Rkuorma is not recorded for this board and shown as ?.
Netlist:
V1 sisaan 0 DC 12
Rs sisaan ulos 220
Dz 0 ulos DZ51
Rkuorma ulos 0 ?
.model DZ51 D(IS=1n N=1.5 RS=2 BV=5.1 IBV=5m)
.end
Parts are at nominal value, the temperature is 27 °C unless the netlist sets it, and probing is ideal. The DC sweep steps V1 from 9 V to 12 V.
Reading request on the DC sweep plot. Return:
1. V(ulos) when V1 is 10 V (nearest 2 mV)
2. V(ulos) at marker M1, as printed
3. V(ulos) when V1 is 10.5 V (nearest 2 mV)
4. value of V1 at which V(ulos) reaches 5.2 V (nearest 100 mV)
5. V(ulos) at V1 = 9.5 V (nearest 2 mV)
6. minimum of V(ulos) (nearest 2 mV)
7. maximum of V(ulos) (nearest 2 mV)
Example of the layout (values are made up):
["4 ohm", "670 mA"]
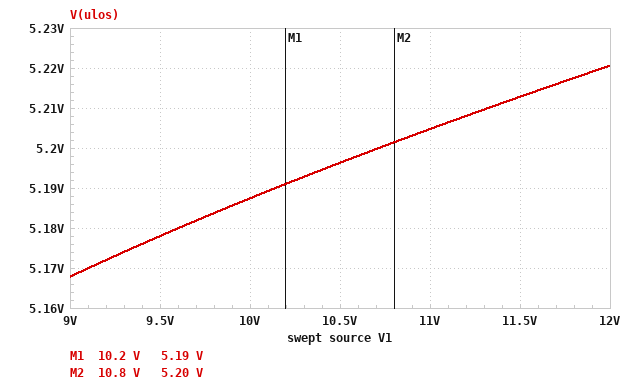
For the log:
["5.188 V", "5.19 V", "5.196 V", "10.7 V", "5.178 V", "5.168 V", "5.220 V"]
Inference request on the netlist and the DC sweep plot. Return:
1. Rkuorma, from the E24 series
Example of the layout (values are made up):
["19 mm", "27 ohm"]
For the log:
["1.5 kΩ"]
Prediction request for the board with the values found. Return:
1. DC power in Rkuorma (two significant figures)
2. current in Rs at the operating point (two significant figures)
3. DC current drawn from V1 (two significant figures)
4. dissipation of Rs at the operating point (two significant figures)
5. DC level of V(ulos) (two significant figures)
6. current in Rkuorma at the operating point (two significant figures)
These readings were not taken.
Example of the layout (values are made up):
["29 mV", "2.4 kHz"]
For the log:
["18 mW", "31 mA", "31 mA", "210 mW", "5.2 V", "3.5 mA"]
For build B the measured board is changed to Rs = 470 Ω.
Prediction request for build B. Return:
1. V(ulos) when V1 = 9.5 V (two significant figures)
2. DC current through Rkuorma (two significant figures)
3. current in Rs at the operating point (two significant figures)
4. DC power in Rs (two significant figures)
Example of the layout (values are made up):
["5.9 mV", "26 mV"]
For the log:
["5.1 V", "3.4 mA", "15 mA", "100 mW"]
